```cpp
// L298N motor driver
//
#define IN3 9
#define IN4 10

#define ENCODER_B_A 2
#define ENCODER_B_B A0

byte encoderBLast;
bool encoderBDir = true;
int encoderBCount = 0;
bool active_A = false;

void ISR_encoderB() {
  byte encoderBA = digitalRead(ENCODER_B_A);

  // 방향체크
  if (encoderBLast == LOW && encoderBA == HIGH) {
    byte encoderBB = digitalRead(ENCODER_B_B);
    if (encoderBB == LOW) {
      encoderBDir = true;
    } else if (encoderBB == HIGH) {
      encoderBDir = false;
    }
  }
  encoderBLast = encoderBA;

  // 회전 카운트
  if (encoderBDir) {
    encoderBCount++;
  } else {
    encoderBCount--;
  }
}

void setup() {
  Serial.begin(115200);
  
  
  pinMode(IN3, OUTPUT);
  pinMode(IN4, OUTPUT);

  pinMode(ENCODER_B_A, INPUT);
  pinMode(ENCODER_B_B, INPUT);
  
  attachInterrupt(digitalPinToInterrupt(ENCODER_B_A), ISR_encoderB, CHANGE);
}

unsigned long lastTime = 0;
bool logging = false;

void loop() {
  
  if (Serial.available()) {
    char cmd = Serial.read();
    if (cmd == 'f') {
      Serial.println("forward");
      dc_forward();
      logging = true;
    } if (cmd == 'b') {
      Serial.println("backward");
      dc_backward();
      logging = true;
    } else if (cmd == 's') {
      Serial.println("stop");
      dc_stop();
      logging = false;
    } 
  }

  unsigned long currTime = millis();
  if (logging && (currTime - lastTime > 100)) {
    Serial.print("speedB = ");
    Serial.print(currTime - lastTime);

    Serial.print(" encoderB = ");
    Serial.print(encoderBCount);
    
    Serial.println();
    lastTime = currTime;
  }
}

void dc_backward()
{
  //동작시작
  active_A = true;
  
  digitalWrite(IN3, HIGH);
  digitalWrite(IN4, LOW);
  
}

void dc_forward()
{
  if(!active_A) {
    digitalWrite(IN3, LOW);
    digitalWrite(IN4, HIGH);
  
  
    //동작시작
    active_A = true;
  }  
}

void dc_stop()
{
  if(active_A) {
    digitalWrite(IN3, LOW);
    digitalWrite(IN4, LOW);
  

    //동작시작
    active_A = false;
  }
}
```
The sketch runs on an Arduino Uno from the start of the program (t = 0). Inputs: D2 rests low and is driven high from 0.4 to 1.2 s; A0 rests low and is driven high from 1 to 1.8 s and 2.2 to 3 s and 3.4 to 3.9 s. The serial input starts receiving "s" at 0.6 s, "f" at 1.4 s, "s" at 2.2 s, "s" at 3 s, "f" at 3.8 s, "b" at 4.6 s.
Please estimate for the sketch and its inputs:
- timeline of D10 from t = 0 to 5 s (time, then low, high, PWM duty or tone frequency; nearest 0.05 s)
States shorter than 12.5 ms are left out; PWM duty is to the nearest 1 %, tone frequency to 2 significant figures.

0 s low; 1.4 s high; 2.2 s low; 3.8 s high; 4.6 s low
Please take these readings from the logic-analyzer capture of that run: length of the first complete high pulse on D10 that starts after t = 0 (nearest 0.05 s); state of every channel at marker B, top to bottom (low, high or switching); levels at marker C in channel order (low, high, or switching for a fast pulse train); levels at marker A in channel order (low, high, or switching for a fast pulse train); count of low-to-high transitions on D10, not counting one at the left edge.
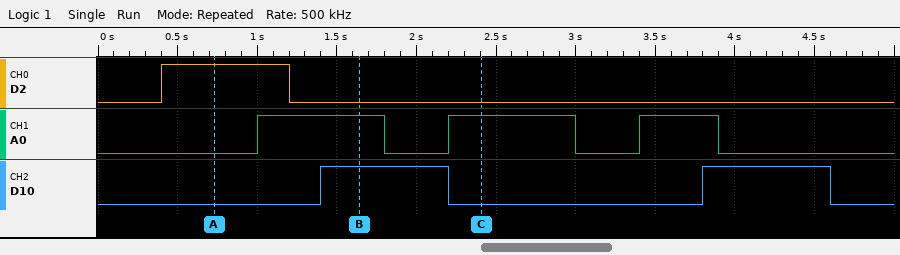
0.80 s
D2 low, A0 high, D10 high
D2 low, A0 high, D10 low
D2 high, A0 low, D10 low
2
